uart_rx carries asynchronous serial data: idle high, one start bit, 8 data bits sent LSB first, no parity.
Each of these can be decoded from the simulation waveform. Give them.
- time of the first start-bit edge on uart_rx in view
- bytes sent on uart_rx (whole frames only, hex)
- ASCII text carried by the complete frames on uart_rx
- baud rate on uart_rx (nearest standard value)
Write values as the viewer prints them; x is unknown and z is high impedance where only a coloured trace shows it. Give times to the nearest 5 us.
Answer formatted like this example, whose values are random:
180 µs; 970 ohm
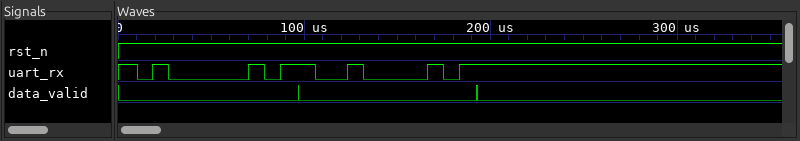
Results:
10 us; 41, 42; "AB"; 115200 baud
